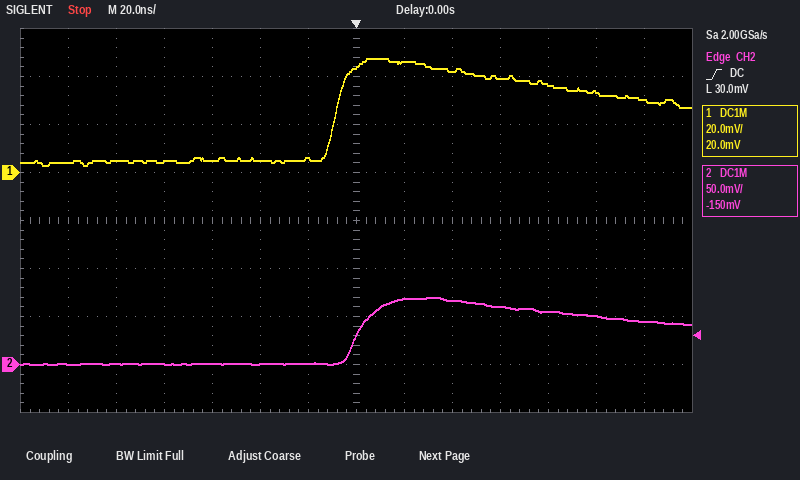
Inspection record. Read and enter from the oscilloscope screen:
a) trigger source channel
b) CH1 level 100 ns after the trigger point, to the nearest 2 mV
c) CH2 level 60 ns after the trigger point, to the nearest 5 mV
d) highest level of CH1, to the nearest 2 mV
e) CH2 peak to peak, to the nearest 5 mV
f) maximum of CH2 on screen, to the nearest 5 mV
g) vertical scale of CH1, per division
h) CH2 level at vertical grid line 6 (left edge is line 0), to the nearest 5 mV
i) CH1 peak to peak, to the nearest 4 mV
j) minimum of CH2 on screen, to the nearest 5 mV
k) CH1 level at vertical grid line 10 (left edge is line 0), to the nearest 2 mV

CH2
34 mV
60 mV
48 mV
70 mV
70 mV
20 mV
0 mV
44 mV
0 mV
40 mV
